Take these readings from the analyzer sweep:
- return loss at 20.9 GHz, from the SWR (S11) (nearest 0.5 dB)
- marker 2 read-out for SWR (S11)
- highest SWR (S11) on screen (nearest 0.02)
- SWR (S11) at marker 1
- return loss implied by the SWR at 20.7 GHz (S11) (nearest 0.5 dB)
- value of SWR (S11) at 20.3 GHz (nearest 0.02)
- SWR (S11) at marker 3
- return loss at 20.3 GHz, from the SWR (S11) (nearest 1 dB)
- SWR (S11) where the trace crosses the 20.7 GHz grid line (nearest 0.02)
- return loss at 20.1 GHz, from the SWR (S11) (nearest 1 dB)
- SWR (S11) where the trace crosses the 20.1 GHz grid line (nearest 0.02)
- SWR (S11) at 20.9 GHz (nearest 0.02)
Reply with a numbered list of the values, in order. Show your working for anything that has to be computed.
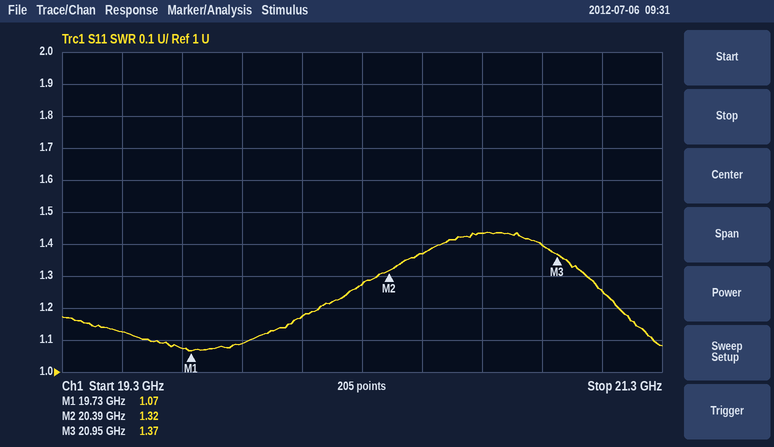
1. −20 log10((1.4 − 1)/(1.4 + 1)) ≈ 15.6 dB, so 15.5 dB to the nearest 0.5 dB
2. 1.32
3. 1.44
4. 1.07
5. −20 log10((1.44 − 1)/(1.44 + 1)) ≈ 14.9 dB, so 15.0 dB to the nearest 0.5 dB
6. 1.28
7. 1.37
8. −20 log10((1.28 − 1)/(1.28 + 1)) ≈ 18 dB
9. 1.44
10. −20 log10((1.18 − 1)/(1.18 + 1)) ≈ 22 dB
11. 1.18
12. 1.40
